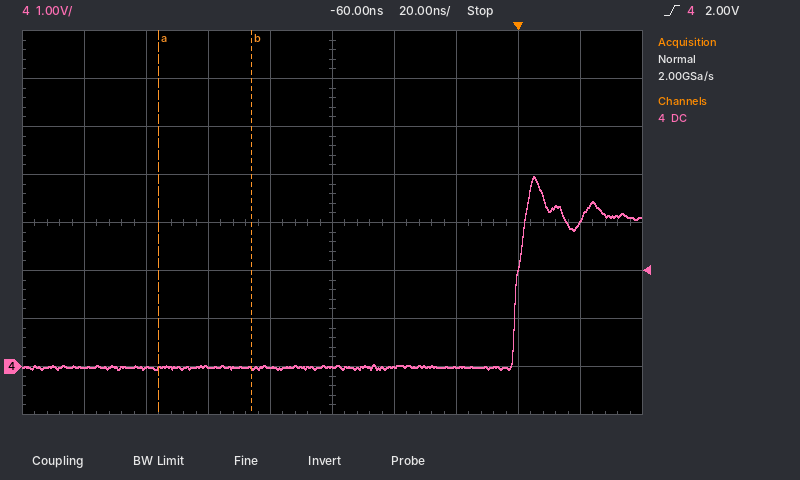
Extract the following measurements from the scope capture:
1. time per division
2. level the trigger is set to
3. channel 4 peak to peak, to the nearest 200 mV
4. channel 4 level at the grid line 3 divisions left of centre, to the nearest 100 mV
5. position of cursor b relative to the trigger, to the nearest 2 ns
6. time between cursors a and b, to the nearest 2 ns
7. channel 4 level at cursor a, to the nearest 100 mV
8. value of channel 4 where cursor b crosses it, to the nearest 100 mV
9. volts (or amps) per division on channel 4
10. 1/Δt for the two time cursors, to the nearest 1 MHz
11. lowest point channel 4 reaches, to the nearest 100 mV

20 ns
2.00 V
4.0 V
0.0 V
-86 ns
30 ns
0.0 V
0.0 V
1 V
33 MHz
-100 mV
